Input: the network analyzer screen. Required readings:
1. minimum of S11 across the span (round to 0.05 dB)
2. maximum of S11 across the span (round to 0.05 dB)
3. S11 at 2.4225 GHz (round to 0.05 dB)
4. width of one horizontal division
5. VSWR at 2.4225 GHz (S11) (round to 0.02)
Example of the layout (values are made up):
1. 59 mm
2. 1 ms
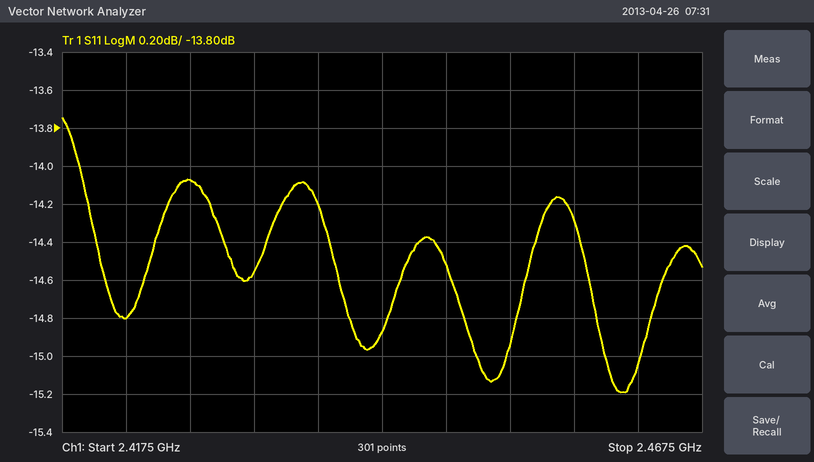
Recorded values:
1. -15.20 dB
2. -13.75 dB
3. -14.80 dB
4. 5 MHz
5. 1.44
